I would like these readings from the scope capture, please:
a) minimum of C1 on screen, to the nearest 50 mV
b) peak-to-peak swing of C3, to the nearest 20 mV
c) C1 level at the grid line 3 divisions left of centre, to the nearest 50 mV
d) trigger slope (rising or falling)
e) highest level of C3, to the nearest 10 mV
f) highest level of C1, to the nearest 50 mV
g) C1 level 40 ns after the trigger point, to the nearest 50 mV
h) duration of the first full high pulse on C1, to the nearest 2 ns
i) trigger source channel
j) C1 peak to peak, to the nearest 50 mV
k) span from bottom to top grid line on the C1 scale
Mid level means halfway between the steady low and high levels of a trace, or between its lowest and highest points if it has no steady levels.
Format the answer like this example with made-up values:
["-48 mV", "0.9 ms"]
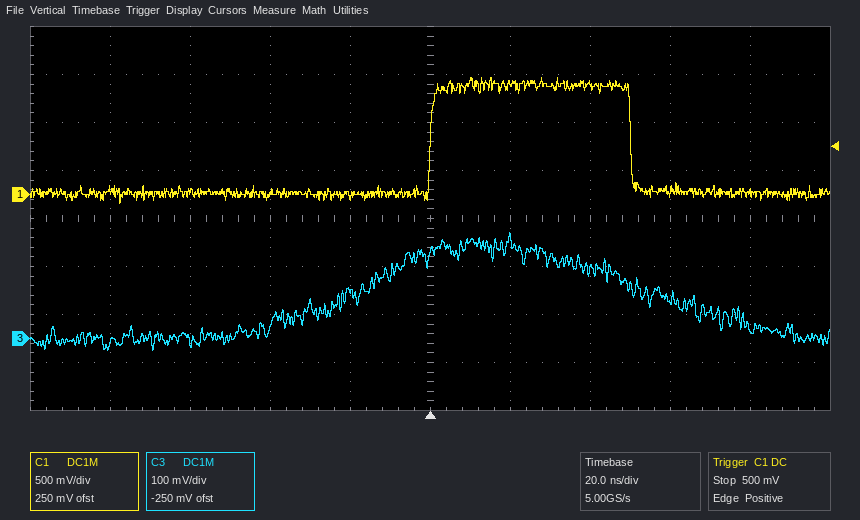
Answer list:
["-100 mV", "240 mV", "0 mV", "rising", "220 mV", "1.20 V", "1.15 V", "50 ns", "C1", "1.30 V", "4 V"]
